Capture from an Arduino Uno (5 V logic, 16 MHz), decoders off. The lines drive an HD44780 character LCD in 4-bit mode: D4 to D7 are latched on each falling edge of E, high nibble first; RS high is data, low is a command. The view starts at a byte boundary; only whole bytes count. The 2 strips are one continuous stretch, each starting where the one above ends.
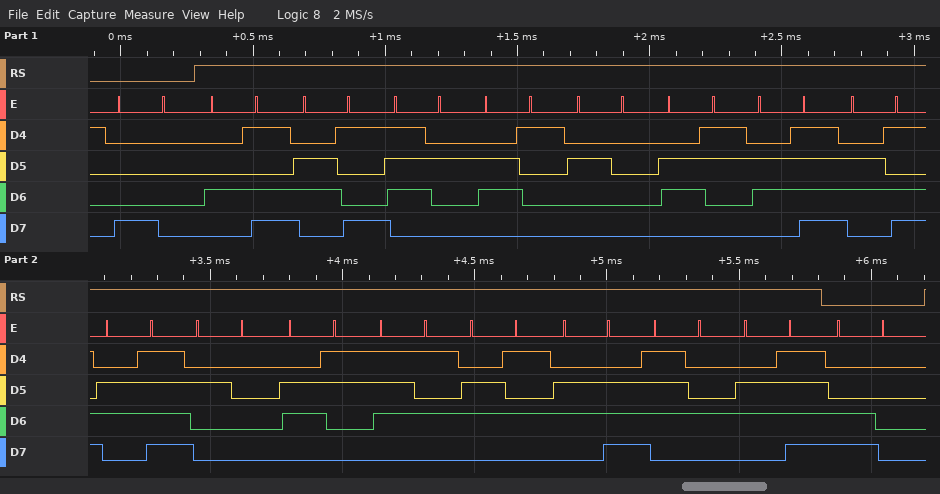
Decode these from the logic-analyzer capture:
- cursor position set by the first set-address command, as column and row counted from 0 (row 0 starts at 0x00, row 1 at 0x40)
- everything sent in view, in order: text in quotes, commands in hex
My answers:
column 0, row 0
0x80 "Mira como cuento" 0xC0
